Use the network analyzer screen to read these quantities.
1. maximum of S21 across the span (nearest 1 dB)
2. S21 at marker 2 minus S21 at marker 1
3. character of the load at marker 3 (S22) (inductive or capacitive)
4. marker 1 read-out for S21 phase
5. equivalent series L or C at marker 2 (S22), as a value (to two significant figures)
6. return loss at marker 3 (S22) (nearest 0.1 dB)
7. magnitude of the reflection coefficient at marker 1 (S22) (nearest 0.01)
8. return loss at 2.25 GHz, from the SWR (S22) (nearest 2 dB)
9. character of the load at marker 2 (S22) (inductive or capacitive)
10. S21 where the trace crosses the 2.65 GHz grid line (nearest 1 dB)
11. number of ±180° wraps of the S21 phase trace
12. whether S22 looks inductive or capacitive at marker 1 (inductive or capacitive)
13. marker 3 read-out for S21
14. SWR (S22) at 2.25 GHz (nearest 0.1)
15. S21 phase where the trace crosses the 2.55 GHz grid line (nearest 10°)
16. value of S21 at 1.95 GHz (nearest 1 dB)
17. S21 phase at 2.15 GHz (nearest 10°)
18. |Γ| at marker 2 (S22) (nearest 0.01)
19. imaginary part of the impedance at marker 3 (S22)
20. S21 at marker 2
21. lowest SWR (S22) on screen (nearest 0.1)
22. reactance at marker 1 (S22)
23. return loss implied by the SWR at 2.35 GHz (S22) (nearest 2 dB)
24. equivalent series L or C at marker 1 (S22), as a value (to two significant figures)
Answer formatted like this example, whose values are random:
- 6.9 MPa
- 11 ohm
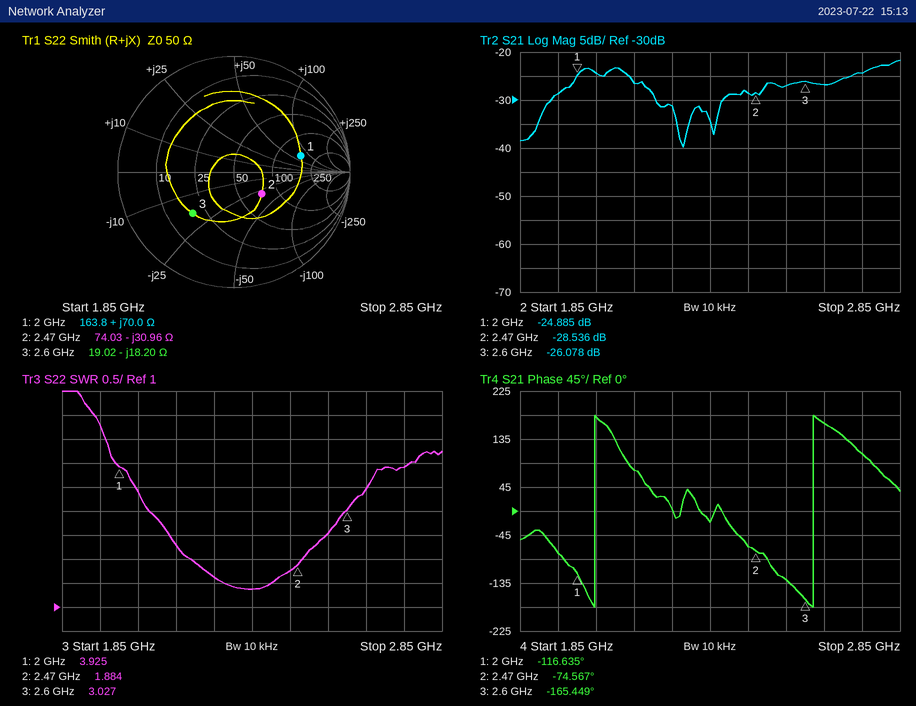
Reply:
- -22 dB
- -3.651 dB
- capacitive
- -116.635°
- 2.1 pF
- 6.0 dB
- 0.59
- 12 dB
- capacitive
- -27 dB
- 2
- inductive
- -26.078 dB
- 1.6
- -130°
- -29 dB
- 80°
- 0.31
- -18.20 Ω
- -28.536 dB
- 1.4
- +70.0 Ω
- 16 dB
- 5.6 nH
